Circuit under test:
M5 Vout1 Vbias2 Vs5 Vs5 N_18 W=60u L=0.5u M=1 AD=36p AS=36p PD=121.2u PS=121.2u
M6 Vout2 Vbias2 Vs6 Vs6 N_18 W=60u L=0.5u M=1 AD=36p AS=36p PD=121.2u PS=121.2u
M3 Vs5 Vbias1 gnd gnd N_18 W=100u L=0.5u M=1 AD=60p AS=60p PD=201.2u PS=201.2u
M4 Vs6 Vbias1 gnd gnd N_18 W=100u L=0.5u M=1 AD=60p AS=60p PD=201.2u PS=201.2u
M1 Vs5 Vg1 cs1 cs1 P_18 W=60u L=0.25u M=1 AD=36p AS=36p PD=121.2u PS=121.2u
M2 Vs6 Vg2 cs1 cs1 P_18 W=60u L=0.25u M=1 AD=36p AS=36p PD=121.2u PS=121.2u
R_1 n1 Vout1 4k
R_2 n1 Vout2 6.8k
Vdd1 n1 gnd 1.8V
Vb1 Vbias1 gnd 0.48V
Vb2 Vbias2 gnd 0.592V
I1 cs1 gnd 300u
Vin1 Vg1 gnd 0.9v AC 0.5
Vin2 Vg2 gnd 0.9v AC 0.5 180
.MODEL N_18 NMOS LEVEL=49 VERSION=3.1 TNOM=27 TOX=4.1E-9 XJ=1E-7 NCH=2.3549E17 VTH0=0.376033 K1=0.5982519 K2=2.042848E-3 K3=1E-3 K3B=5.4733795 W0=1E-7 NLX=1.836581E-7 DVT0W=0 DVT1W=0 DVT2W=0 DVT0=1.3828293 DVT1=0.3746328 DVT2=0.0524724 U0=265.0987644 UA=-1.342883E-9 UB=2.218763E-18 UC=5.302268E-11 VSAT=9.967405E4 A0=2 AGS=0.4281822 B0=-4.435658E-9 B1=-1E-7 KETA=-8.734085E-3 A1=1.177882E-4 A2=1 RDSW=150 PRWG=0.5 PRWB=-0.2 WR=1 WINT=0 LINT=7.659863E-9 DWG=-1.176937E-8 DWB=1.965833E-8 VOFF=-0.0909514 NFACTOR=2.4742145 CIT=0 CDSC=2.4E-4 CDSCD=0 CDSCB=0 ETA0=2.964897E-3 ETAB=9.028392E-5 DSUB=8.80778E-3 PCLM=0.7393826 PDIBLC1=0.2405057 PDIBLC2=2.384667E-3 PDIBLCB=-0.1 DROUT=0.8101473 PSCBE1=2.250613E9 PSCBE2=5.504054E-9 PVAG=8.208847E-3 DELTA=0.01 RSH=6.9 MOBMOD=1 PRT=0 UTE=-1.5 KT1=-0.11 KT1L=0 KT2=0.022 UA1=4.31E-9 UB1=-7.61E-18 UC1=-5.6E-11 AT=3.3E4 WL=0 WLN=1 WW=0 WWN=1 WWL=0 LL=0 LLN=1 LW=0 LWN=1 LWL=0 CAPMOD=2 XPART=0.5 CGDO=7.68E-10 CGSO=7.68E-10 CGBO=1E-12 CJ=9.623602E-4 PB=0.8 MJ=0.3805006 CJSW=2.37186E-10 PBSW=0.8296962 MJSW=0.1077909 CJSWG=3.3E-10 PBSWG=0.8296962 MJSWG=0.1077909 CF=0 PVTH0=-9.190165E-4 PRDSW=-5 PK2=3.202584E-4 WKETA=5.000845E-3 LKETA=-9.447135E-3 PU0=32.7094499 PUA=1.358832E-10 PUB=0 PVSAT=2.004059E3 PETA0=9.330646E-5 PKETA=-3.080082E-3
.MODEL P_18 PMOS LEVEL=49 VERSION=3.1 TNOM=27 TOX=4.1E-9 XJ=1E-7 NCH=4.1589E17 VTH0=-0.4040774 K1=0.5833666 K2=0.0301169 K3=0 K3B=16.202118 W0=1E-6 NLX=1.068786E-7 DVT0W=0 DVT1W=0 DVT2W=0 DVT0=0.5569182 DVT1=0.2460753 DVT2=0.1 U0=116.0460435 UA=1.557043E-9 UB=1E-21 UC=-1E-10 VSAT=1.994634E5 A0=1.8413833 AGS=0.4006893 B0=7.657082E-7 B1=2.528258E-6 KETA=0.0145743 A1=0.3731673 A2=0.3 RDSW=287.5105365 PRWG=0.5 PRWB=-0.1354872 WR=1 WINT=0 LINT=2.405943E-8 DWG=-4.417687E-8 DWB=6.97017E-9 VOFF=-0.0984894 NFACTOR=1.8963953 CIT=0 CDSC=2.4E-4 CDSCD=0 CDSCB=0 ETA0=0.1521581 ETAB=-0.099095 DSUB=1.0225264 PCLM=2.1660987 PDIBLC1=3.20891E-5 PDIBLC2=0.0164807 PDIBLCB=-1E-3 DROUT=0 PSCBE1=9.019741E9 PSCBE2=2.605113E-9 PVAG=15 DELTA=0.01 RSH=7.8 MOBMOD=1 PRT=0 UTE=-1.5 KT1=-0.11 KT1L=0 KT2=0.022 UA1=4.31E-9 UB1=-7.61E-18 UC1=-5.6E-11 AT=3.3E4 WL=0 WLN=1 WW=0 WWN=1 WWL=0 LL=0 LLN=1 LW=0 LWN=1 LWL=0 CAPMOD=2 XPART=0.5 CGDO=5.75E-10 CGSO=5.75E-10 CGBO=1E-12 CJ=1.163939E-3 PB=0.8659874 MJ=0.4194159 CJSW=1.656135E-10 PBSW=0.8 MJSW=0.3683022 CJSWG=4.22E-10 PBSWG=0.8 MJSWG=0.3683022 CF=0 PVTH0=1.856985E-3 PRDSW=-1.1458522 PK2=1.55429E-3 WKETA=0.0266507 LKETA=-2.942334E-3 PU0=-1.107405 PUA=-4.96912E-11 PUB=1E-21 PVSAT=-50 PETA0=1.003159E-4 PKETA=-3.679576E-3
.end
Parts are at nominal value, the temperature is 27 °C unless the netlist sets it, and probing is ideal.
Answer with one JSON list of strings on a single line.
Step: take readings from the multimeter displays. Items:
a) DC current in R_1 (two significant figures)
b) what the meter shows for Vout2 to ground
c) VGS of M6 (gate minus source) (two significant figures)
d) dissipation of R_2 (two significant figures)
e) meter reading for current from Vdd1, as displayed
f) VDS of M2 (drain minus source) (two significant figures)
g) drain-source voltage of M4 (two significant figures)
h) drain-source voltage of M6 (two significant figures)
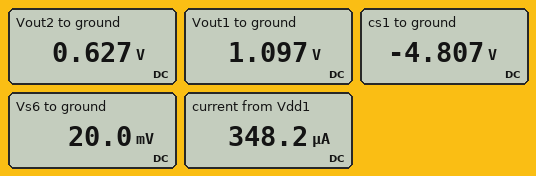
["180 µA", "0.627 V", "570 mV", "200 µW", "348.2 µA", "4.8 V", "20 mV", "610 mV"]
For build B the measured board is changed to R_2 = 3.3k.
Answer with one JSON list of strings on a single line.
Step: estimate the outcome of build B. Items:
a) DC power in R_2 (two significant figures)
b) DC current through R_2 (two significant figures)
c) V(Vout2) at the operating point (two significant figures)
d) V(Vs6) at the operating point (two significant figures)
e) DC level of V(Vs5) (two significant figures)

["100 µW", "180 µA", "1.2 V", "25 mV", "24 mV"]
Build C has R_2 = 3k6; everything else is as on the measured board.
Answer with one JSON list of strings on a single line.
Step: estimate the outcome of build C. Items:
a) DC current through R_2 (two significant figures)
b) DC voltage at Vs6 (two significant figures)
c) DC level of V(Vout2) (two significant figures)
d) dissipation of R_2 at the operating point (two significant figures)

["180 µA", "24 mV", "1.2 V", "110 µW"]
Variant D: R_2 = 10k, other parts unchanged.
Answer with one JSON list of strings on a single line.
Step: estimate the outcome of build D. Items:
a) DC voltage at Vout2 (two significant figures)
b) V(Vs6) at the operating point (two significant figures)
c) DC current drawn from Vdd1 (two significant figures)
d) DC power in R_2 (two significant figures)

["140 mV", "13 mV", "340 µA", "280 µW"]
